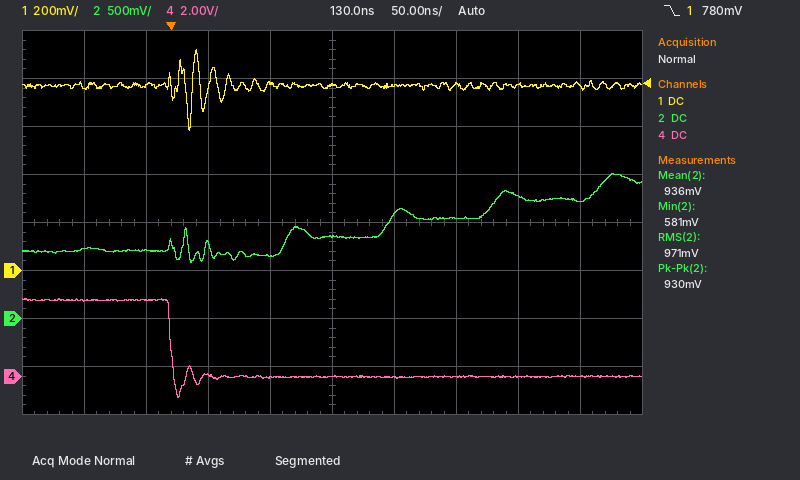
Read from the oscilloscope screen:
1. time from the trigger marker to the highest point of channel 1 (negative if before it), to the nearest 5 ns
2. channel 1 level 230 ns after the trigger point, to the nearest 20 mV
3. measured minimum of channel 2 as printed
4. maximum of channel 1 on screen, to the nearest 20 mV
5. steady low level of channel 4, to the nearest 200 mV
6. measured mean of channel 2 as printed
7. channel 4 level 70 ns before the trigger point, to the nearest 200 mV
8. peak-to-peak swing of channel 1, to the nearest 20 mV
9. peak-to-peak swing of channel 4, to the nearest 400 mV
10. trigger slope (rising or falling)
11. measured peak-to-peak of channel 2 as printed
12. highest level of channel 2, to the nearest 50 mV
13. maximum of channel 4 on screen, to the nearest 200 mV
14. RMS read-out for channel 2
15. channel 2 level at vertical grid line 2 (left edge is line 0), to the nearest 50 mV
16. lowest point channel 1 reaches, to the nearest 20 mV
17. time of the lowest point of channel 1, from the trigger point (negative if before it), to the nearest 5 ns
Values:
+20 ns
780 mV
581 mV
920 mV
0.0 V
936 mV
3.2 V
340 mV
4.0 V
falling
930 mV
1.50 V
3.2 V
971 mV
700 mV
580 mV
+15 ns
